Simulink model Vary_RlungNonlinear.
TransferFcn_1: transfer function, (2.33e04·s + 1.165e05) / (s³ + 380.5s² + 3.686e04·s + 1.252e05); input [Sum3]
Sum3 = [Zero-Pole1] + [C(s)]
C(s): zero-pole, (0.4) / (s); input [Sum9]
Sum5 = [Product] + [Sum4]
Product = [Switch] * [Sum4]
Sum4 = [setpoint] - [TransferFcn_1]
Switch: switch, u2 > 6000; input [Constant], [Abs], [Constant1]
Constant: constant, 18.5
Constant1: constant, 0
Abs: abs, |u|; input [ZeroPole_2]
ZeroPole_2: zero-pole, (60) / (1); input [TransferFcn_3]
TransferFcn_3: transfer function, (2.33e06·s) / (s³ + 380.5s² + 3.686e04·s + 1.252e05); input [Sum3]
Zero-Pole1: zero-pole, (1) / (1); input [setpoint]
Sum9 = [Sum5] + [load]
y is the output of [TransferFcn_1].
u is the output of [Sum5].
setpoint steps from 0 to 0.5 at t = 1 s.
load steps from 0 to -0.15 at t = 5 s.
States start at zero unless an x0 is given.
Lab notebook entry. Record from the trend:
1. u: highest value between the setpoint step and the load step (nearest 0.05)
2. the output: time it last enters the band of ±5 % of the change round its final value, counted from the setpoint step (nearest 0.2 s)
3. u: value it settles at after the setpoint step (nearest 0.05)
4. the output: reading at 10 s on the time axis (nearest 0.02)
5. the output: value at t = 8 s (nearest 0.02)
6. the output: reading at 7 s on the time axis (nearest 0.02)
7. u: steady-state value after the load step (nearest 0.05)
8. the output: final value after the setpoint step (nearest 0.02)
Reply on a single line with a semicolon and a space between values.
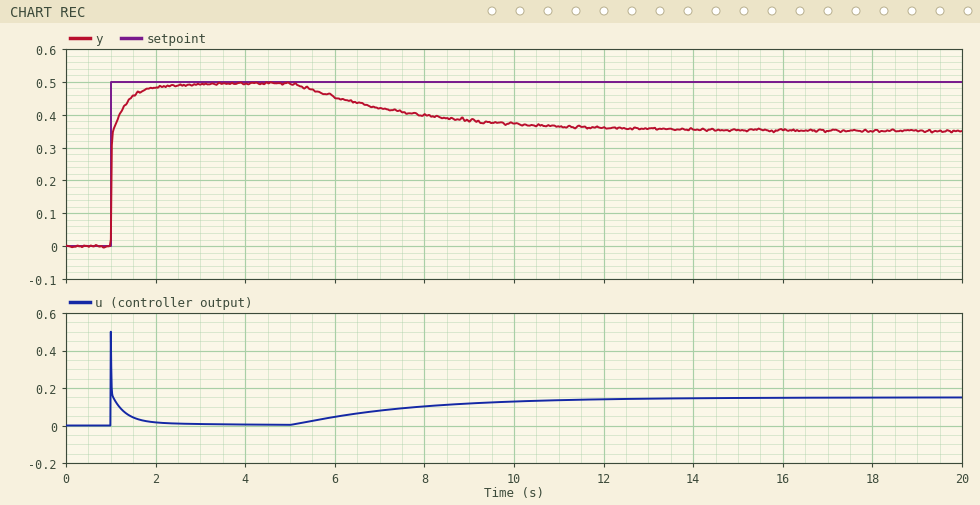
0.50; 0.8 s; 0.00; 0.38; 0.40; 0.42; 0.15; 0.50
